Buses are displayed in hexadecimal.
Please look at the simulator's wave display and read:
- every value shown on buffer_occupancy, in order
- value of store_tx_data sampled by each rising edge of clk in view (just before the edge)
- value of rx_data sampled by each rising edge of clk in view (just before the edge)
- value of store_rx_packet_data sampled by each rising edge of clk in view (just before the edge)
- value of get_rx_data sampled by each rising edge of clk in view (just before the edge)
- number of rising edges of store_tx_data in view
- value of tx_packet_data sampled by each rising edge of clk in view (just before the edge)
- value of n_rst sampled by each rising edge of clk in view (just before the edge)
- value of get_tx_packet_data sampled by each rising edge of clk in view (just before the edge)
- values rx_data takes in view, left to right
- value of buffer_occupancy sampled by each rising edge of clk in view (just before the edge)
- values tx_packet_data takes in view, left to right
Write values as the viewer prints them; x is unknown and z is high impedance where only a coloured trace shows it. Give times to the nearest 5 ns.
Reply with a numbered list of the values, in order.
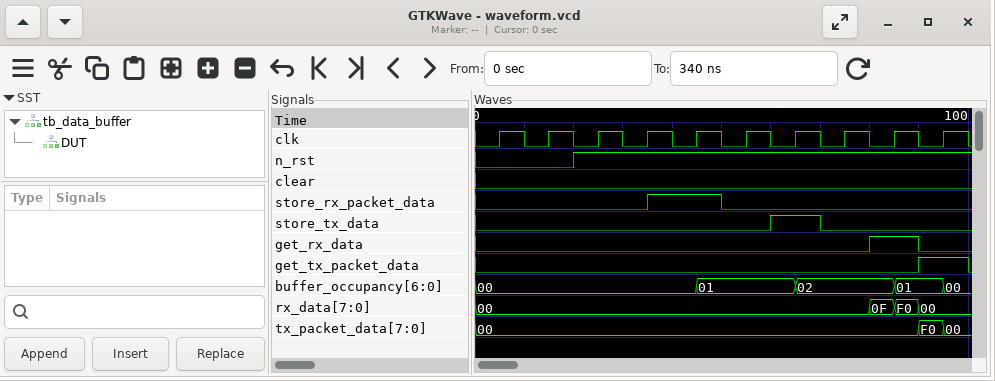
1. 00, 01, 02, 01, 00
2. 0 0 0 0 0 0 1 0 0 0
3. 00, 00, 00, 00, 00, 00, 00, 00, 0F, 00
4. 0 0 0 0 1 0 0 0 0 0
5. 0 0 0 0 0 0 0 0 1 0
6. 1
7. 00, 00, 00, 00, 00, 00, 00, 00, 00, F0
8. 0 0 1 1 1 1 1 1 1 1
9. 0 0 0 0 0 0 0 0 0 1
10. 00, 0F, F0, 00
11. 00, 00, 00, 00, 00, 01, 01, 02, 02, 01
12. 00, F0, 00
